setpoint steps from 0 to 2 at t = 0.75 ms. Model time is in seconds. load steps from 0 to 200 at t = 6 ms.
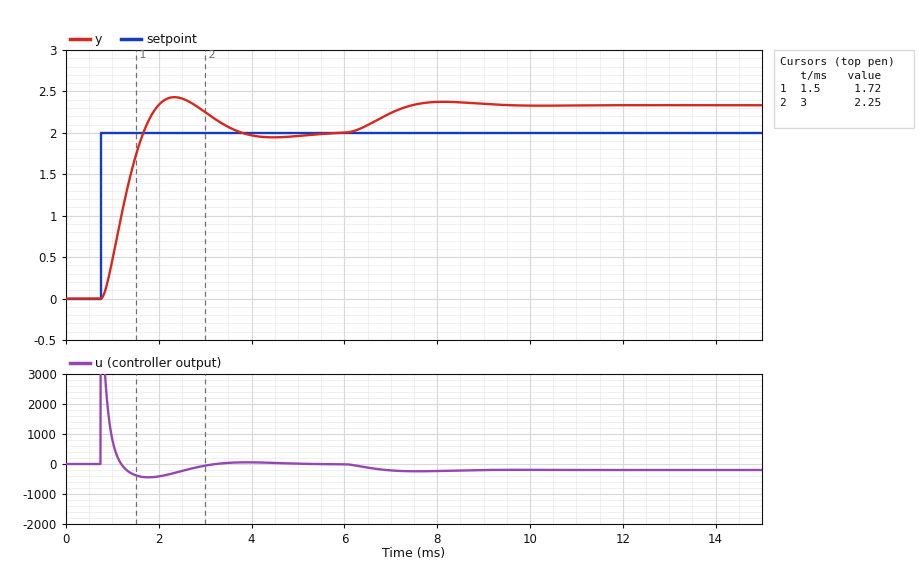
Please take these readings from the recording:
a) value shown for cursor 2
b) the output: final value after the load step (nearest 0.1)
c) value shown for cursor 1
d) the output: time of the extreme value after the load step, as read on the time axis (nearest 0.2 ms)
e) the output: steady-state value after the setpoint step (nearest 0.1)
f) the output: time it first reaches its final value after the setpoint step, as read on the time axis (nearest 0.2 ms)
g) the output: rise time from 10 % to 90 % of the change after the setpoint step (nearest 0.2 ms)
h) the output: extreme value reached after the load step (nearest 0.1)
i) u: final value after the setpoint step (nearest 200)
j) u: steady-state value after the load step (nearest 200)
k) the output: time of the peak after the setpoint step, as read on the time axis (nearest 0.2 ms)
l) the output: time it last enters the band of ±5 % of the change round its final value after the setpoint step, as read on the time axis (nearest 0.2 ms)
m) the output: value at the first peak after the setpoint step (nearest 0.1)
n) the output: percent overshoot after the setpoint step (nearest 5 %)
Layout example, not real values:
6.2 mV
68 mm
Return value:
2.25
2.3
1.72
8.2 ms
2.0
1.6 ms
0.6 ms
2.4
0
-200
2.4 ms
3.4 ms
2.4
20 %
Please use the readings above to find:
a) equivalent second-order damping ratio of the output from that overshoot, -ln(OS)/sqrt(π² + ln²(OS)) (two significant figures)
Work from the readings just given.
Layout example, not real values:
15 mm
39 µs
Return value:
0.46
